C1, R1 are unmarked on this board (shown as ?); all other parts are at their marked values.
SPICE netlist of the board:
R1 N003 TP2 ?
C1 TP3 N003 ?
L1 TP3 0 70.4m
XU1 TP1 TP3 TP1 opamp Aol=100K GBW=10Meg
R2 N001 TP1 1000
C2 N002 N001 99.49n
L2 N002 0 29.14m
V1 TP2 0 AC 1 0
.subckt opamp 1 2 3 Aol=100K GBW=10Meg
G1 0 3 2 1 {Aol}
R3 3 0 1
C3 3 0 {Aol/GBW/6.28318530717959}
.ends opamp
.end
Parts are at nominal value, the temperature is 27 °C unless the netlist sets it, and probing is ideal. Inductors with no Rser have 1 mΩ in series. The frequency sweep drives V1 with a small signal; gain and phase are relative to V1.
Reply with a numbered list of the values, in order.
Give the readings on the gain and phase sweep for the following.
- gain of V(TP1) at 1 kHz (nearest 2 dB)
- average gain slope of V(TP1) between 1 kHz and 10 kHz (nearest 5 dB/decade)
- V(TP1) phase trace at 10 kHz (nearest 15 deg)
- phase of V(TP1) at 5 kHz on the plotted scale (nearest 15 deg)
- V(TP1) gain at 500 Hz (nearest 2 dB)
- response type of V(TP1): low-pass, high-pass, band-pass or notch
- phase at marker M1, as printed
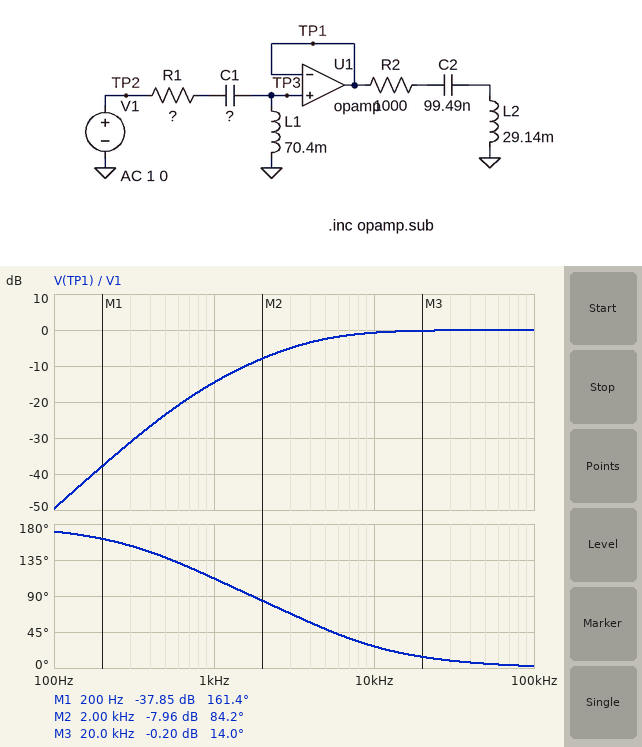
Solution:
1. -14 dB
2. 15 dB/decade
3. 30 deg
4. 45 deg
5. -24 dB
6. high-pass
7. 161.4 deg
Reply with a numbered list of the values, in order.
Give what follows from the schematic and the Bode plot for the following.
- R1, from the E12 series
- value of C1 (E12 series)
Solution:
1. 2.2 kΩ
2. 120 nF
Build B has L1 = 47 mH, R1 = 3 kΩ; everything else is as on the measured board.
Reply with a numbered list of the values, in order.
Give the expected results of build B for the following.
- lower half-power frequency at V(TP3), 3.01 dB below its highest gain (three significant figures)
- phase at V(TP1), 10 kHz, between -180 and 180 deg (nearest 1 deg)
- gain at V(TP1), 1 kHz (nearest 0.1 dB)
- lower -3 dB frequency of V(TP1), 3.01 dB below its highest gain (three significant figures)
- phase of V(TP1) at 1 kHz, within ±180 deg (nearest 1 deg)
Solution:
1. 9.72 kHz
2. 47 deg
3. -20.6 dB
4. 9.70 kHz
5. 109 deg
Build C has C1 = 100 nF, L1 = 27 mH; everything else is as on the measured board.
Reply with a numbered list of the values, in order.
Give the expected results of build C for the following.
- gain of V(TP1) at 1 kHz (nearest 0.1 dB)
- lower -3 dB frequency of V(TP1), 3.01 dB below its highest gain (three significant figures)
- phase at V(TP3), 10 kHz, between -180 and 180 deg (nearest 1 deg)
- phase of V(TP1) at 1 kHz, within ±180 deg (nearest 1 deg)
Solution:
1. -23.8 dB
2. 12.2 kHz
3. 55 deg
4. 123 deg
